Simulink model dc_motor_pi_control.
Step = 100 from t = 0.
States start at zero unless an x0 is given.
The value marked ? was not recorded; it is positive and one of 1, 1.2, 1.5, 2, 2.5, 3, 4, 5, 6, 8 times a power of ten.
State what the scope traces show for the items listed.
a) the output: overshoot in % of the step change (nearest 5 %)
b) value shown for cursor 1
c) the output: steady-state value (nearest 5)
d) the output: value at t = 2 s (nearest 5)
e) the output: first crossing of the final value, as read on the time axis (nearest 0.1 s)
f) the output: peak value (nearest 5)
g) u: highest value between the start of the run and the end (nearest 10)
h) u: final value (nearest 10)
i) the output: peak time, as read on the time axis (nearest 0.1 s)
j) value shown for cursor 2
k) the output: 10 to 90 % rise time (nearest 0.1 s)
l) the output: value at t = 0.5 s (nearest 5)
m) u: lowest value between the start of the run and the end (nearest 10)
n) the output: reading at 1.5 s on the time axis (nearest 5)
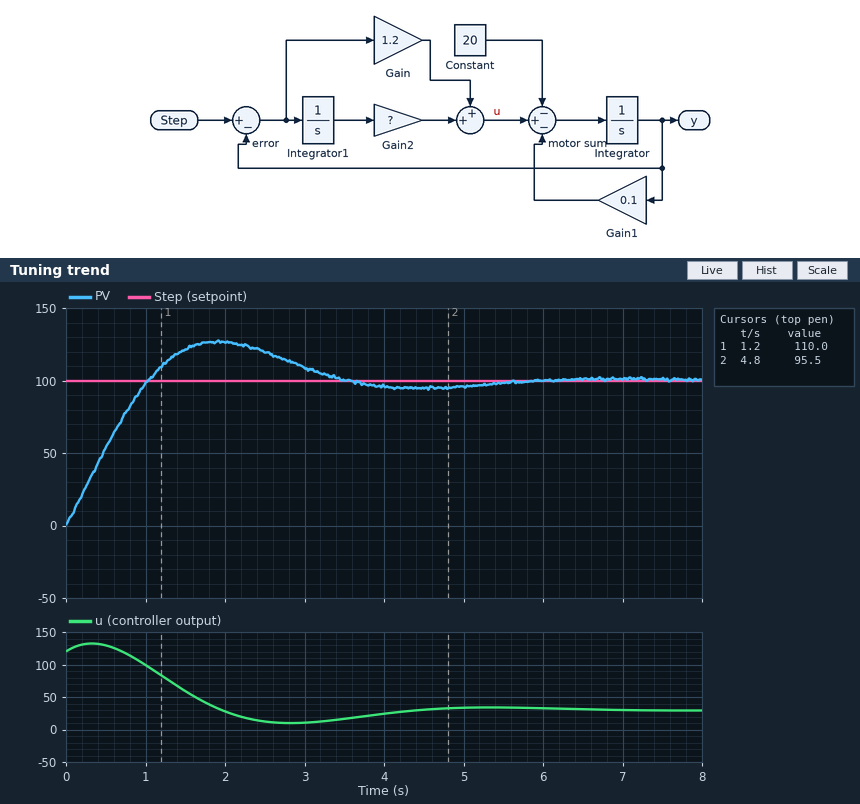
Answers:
25 %
110.0
100
125
1.0 s
125
130
30
1.9 s
95.5
0.8 s
55
10
120
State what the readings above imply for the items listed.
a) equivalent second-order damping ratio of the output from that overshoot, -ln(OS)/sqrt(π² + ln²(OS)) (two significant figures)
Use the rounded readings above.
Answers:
0.40
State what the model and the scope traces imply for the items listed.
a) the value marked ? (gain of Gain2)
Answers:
2
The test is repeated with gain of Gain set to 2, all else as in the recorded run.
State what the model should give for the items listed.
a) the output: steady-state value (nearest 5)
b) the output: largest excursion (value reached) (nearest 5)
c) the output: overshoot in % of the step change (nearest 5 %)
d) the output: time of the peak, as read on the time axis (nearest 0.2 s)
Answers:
100
115
15 %
1.8 s
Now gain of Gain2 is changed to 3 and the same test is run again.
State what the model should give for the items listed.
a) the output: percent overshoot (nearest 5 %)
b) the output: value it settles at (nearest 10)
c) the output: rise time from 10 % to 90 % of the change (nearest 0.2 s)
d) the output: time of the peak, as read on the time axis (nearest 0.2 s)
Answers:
35 %
100
0.6 s
1.6 s
